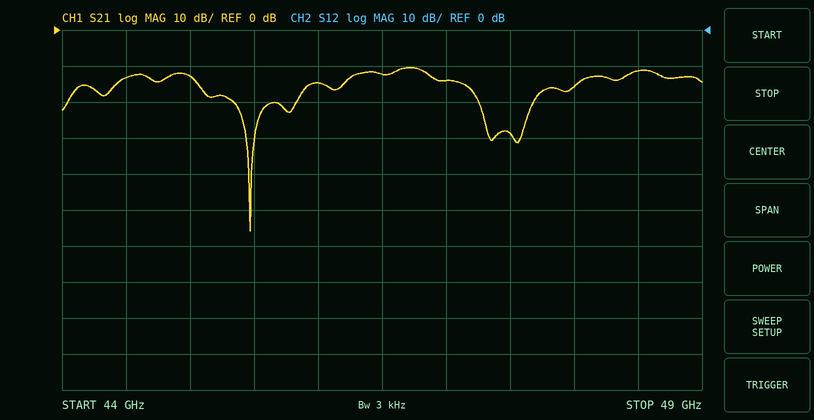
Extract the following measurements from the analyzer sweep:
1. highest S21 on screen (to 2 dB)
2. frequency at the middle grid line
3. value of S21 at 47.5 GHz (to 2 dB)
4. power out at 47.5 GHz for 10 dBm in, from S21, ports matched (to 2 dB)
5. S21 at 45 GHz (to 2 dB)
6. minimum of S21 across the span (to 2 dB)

-10 dB
46.5 GHz
-28 dB
-18 dBm
-12 dB
-56 dB
